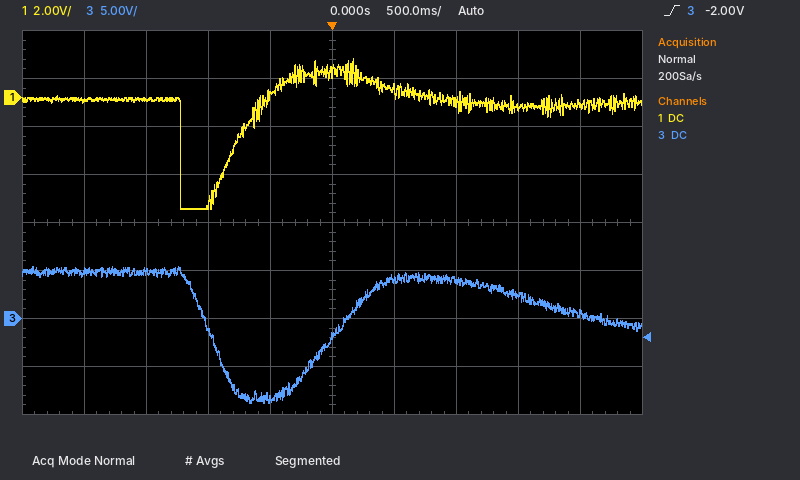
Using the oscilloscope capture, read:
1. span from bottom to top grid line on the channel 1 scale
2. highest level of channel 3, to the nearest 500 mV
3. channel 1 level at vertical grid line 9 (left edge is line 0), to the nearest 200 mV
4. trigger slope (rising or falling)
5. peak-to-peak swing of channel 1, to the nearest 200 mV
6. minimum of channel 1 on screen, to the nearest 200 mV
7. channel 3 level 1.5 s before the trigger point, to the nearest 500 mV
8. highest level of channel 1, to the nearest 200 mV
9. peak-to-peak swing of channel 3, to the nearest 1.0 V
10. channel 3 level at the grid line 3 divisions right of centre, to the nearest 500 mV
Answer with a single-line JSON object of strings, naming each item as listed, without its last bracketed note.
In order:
{"span from bottom to top grid line on the channel 1 scale": "16 V", "highest level of channel 3, to the nearest 500 mV": "5.5 V", "channel 1 level at vertical grid line 9 (left edge is line 0), to the nearest 200 mV": "-200 mV", "trigger slope": "rising", "peak-to-peak swing of channel 1, to the nearest 200 mV": "6.2 V", "minimum of channel 1 on screen, to the nearest 200 mV": "-4.6 V", "channel 3 level 1.5 s before the trigger point, to the nearest 500 mV": "5.0 V", "highest level of channel 1, to the nearest 200 mV": "1.6 V", "peak-to-peak swing of channel 3, to the nearest 1.0 V": "14.0 V", "channel 3 level at the grid line 3 divisions right of centre, to the nearest 500 mV": "2.5 V"}
